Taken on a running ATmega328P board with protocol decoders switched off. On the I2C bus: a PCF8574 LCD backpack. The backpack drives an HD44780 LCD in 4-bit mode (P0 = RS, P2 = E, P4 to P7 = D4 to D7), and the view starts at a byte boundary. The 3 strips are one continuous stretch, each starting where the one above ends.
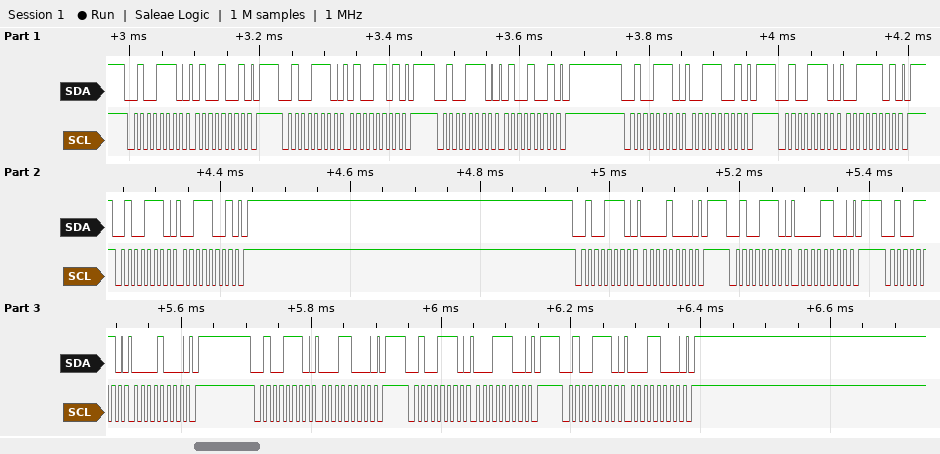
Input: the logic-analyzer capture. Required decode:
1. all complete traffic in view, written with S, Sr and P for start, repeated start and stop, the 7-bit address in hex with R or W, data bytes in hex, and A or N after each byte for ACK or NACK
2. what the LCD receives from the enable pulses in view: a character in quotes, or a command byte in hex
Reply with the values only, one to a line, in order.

S 27W A 49 A P S 27W A 4D A P S 27W A 49 A P S 27W A 39 A P S 27W A 3D A P S 27W A 39 A P S 27W A 08 A P S 27W A 0C A P S 27W A 08 A P S 27W A 18 A P S 27W A 1C A P S 27W A 18 A P
'C' 0x01
